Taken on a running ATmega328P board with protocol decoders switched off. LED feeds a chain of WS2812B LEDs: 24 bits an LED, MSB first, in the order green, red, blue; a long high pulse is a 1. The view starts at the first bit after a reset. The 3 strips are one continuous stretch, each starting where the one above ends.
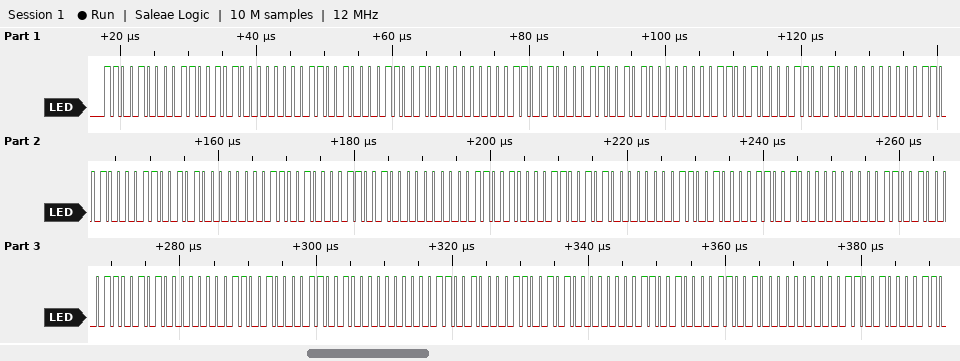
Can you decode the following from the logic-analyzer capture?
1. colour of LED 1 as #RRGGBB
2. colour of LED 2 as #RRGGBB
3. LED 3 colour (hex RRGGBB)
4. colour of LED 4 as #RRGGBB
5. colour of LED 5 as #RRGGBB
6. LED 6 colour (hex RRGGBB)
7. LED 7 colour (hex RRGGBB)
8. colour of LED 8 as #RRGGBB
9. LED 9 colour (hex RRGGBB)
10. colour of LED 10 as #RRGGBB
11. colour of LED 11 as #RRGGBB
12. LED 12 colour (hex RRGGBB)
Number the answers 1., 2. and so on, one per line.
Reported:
1. #65C800
2. #64C800
3. #65C800
4. #64C800
5. #65C800
6. #64C800
7. #65C800
8. #64C800
9. #65C800
10. #64C800
11. #65C800
12. #64C800
